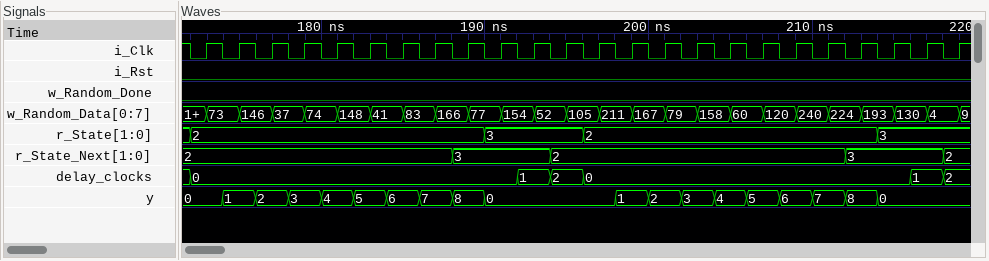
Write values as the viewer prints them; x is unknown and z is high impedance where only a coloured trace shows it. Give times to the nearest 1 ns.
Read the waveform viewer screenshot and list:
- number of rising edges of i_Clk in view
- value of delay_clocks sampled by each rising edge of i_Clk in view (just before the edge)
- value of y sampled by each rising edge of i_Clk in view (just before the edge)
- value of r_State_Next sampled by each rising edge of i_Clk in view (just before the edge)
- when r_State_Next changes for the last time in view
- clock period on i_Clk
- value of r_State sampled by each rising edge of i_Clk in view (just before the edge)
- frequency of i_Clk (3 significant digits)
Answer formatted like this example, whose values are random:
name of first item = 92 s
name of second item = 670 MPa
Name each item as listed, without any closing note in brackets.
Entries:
number of rising edges of i_Clk in view = 24
value of delay_clocks sampled by each rising edge of i_Clk in view = 0, 0, 0, 0, 0, 0, 0, 0, 0, 0, 1, 2, 0, 0, 0, 0, 0, 0, 0, 0, 0, 0, 1, 2
value of y sampled by each rising edge of i_Clk in view = 0, 1, 2, 3, 4, 5, 6, 7, 8, 0, 0, 0, 0, 1, 2, 3, 4, 5, 6, 7, 8, 0, 0, 0
value of r_State_Next sampled by each rising edge of i_Clk in view = 2, 2, 2, 2, 2, 2, 2, 2, 3, 3, 3, 2, 2, 2, 2, 2, 2, 2, 2, 2, 3, 3, 3, 2
when r_State_Next changes for the last time in view = 218 ns
clock period on i_Clk = 2 ns
value of r_State sampled by each rising edge of i_Clk in view = 2, 2, 2, 2, 2, 2, 2, 2, 2, 3, 3, 3, 2, 2, 2, 2, 2, 2, 2, 2, 2, 3, 3, 3
frequency of i_Clk = 500 MHz
